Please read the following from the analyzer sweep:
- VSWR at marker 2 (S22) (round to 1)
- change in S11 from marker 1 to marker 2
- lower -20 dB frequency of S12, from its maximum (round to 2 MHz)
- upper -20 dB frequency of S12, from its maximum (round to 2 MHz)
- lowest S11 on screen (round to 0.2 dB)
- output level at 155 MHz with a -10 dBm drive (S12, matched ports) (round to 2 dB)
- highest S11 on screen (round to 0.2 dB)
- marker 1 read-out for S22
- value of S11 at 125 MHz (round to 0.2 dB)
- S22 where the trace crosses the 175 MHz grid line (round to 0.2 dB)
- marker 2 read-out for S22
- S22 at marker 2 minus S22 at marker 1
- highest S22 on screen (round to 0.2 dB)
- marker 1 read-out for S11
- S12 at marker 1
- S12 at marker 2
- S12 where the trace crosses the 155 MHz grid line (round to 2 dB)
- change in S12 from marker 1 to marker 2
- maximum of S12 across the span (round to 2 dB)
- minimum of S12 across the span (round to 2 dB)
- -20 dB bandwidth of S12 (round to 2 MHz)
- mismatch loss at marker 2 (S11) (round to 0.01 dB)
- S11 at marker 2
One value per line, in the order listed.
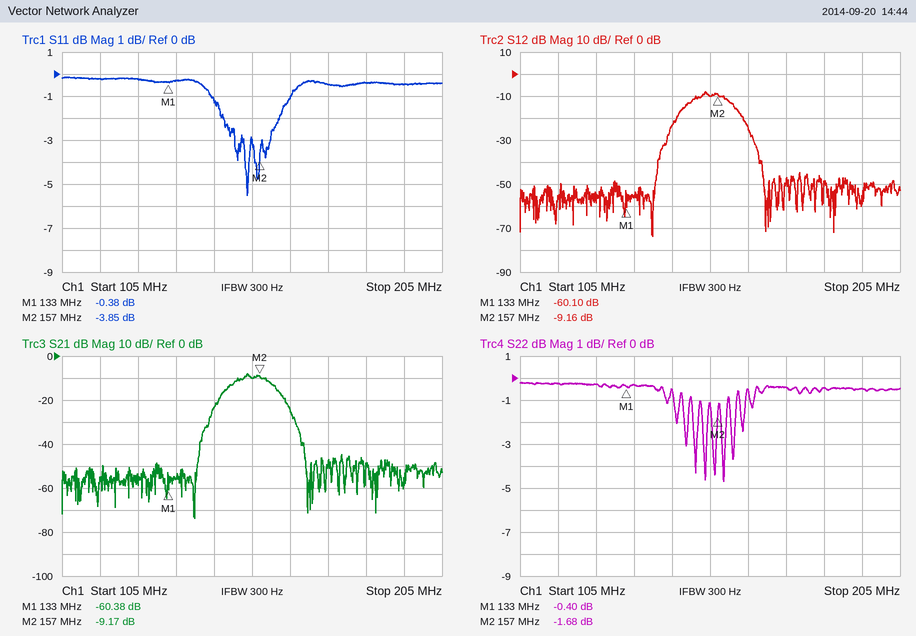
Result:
10
-3.47 dB
144 MHz
166 MHz
-5.6 dB
-20 dBm
-0.2 dB
-0.40 dB
-0.2 dB
-0.4 dB
-1.68 dB
-1.28 dB
-0.2 dB
-0.38 dB
-60.10 dB
-9.16 dB
-10 dB
50.94 dB
-8 dB
-74 dB
22 MHz
2.31 dB
-3.85 dB
